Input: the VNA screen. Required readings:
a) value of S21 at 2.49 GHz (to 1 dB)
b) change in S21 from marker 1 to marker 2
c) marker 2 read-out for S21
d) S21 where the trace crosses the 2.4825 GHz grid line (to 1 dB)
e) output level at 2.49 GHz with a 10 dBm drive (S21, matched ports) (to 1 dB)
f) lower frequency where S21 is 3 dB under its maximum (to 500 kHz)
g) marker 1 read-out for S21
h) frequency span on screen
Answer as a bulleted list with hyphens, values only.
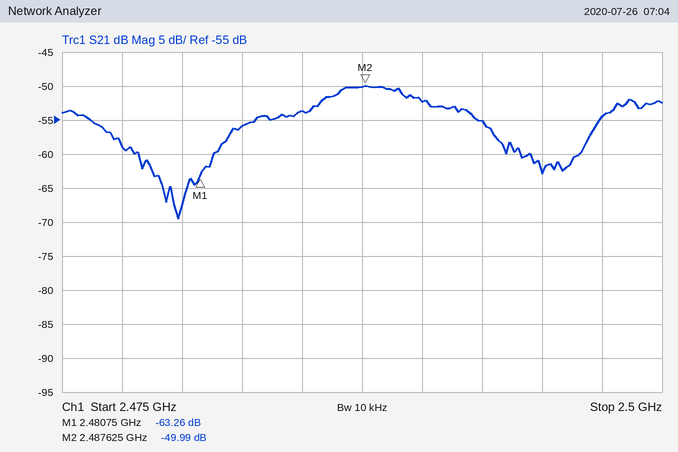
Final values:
- -52 dB
- 13.27 dB
- -49.99 dB
- -56 dB
- -42 dBm
- 2.4855 GHz
- -63.26 dB
- 25 MHz
